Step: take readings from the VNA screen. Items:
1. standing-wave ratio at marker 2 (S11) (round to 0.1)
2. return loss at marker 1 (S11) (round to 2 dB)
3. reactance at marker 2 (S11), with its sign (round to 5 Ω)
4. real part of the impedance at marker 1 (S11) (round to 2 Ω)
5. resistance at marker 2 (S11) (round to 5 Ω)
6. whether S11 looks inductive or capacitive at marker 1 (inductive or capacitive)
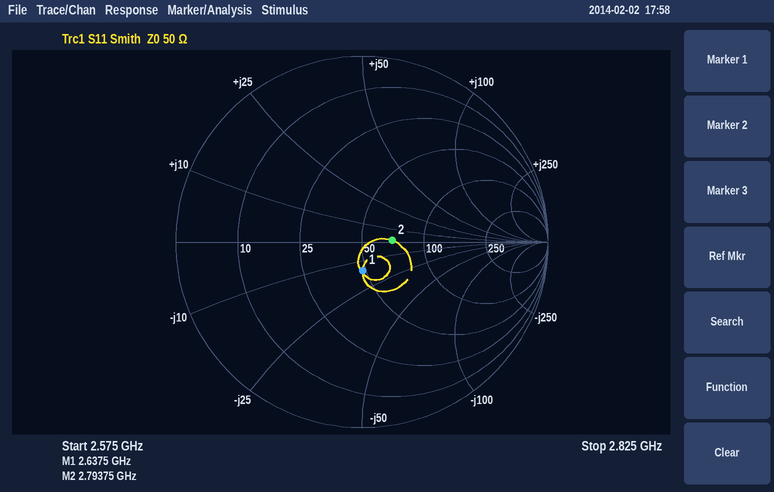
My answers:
1.4
16 dB
0 Ω
48 Ω
70 Ω
capacitive
